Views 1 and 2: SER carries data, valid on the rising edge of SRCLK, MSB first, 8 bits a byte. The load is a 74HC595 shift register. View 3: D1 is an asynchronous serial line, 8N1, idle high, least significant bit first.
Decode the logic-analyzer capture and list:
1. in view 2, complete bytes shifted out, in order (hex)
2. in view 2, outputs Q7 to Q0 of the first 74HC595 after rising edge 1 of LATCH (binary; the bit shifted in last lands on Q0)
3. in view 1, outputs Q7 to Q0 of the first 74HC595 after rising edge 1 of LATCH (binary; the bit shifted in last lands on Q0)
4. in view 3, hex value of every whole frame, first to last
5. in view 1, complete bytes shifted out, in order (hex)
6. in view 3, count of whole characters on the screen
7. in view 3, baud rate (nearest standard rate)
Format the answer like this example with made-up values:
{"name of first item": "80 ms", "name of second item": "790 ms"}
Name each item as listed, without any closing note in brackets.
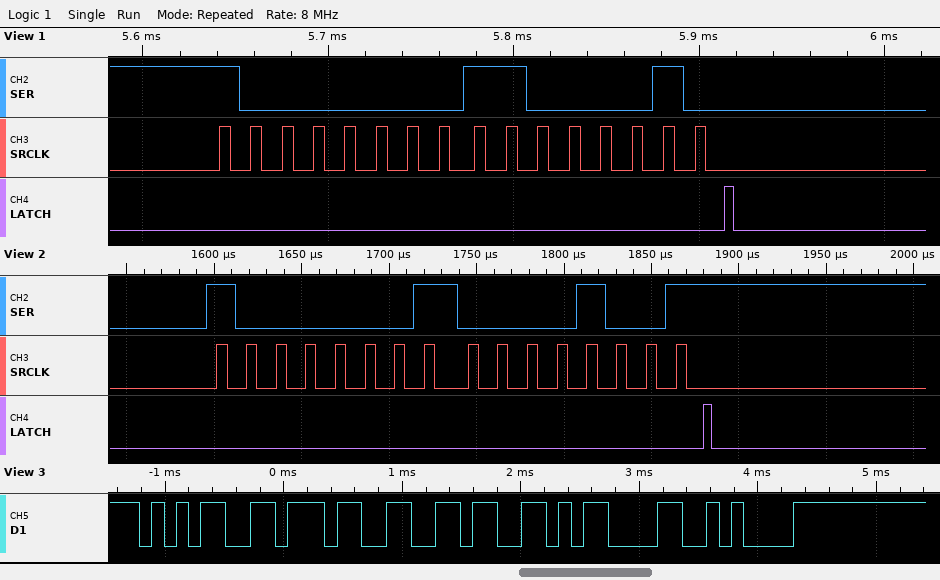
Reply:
{"in view 2, complete bytes shifted out, in order": "81 09", "in view 2, outputs Q7 to Q0 of the first 74HC595 after rising edge 1 of LATCH": "00001001", "in view 1, outputs Q7 to Q0 of the first 74HC595 after rising edge 1 of LATCH": "11000010", "in view 3, hex value of every whole frame, first to last": "35 37 36 0D 0A", "in view 1, complete bytes shifted out, in order": "80 C2", "in view 3, count of whole characters on the screen": "5", "in view 3, baud rate": "9600 baud"}
